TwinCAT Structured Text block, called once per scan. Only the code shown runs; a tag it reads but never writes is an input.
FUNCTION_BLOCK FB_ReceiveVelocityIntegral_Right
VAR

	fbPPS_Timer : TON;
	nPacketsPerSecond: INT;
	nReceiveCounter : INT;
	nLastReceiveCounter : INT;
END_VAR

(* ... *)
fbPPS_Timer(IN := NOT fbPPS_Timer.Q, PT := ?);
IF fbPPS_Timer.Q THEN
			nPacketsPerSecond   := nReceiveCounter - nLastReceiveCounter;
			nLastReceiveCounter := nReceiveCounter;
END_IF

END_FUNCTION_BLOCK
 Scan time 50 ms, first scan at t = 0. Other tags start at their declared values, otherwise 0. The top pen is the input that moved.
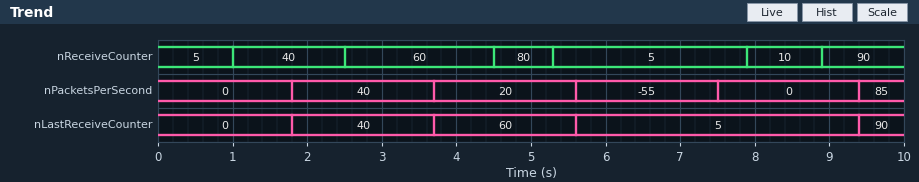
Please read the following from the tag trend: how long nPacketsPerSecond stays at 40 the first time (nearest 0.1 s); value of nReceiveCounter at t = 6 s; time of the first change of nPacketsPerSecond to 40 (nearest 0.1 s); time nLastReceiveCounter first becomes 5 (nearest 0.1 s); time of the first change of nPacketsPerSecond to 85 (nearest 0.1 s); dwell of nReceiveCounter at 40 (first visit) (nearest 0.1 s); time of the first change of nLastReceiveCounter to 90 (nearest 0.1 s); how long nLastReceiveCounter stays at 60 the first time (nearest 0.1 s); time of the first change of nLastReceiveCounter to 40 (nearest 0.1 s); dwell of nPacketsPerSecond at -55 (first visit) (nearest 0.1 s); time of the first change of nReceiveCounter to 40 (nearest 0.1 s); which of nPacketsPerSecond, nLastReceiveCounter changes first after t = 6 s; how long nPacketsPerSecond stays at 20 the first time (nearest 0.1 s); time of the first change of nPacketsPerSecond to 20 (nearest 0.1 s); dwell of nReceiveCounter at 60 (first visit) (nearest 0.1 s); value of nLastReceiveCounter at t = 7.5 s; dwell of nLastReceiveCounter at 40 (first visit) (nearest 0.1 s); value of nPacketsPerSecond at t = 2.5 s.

1.9 s
5
1.8 s
5.6 s
9.4 s
1.5 s
9.4 s
1.9 s
1.8 s
1.9 s
1.0 s
nPacketsPerSecond
1.9 s
3.7 s
2.0 s
5
1.9 s
40
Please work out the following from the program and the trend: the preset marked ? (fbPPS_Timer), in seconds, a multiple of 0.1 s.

1.8 s
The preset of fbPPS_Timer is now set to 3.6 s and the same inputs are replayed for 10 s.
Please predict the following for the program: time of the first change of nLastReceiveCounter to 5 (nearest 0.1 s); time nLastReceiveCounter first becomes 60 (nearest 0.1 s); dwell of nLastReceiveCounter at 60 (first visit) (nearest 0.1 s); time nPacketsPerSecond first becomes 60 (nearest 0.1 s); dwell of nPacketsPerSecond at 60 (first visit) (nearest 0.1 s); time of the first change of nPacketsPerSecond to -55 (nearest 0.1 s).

7.3 s
3.6 s
3.7 s
3.6 s
3.7 s
7.3 s
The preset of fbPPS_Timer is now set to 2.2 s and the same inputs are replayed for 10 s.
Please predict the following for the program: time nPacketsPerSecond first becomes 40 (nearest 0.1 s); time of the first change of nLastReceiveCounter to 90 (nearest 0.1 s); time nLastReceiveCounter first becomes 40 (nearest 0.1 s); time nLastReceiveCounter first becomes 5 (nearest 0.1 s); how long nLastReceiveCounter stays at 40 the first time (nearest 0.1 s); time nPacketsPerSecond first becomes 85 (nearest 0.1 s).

2.2 s
9.1 s
2.2 s
6.8 s
2.3 s
9.1 s
